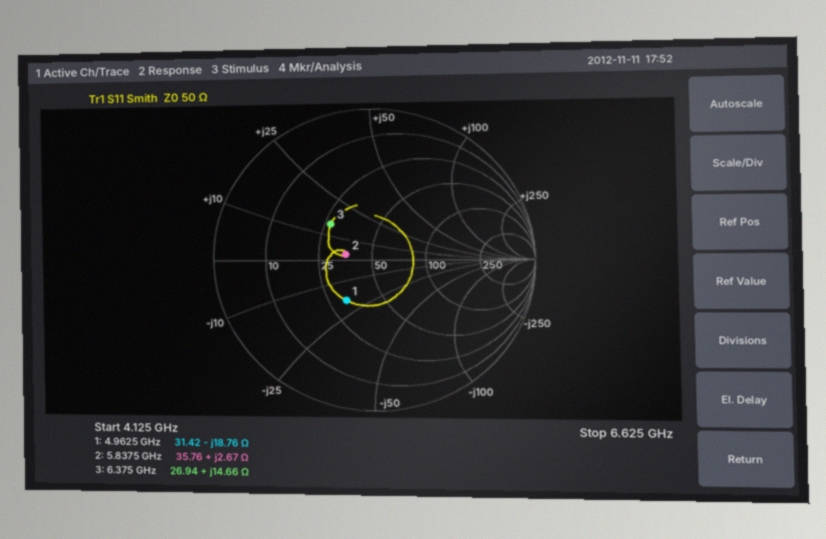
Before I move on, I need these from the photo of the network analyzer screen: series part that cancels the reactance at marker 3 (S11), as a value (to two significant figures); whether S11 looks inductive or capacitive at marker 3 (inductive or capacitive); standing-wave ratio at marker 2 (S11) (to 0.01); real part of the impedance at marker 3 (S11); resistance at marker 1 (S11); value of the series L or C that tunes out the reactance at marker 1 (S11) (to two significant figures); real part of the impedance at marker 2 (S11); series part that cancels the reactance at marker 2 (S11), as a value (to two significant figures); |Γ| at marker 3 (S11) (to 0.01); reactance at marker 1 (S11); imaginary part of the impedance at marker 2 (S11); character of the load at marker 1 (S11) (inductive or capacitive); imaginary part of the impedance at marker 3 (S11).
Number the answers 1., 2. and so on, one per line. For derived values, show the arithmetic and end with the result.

1. C = 1/(2π × 6.375 GHz × 14.66 Ω) ≈ 1.7 pF
2. inductive
3. 1.41
4. 26.94 Ω
5. 31.42 Ω
6. L = 18.76 Ω/(2π × 4.9625 GHz) ≈ 602 pH, so 600 pH to two significant figures
7. 35.76 Ω
8. C = 1/(2π × 5.8375 GHz × 2.67 Ω) ≈ 10 pF
9. 0.35
10. -18.76 Ω
11. +2.67 Ω
12. capacitive
13. +14.66 Ω
